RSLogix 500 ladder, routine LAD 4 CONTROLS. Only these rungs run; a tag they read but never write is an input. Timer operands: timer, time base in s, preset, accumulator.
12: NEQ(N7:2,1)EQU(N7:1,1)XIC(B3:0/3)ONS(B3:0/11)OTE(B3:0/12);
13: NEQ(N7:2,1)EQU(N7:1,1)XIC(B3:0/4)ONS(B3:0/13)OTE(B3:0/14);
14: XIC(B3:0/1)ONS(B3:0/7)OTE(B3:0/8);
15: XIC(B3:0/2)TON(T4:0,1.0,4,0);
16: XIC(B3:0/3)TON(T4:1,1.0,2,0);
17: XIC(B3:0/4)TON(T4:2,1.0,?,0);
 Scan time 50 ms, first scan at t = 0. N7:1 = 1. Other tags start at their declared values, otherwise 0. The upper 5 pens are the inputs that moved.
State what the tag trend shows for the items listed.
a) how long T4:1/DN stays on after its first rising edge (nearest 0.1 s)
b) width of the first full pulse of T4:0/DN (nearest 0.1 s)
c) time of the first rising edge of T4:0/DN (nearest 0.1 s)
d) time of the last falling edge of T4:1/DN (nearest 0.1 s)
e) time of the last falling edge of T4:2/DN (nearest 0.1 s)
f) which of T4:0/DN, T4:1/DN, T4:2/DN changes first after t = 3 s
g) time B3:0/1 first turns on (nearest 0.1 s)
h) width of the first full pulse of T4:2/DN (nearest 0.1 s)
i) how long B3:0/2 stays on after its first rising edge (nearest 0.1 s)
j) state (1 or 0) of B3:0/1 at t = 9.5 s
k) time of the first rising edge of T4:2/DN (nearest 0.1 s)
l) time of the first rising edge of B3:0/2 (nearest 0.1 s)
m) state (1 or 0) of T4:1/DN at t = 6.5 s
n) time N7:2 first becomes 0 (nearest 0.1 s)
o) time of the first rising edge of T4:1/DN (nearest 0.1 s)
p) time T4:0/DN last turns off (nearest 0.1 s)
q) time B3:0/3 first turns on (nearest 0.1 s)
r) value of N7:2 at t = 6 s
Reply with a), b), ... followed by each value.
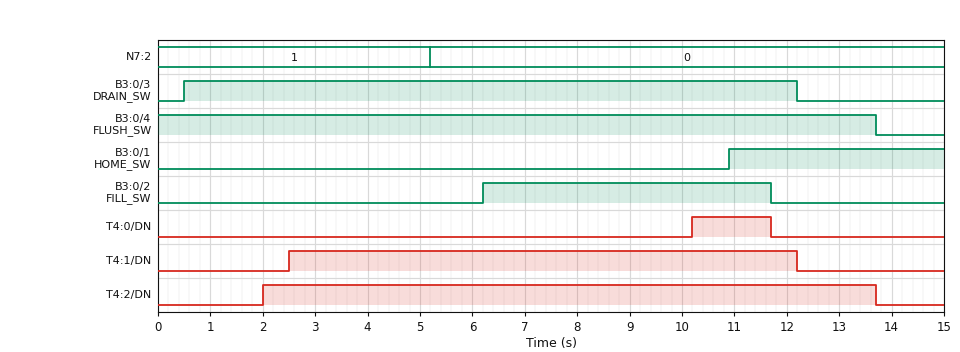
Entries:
a) 9.7 s
b) 1.5 s
c) 10.2 s
d) 12.2 s
e) 13.7 s
f) T4:0/DN
g) 10.9 s
h) 11.7 s
i) 5.5 s
j) 0
k) 2.0 s
l) 6.2 s
m) 1
n) 5.2 s
o) 2.5 s
p) 11.7 s
q) 0.5 s
r) 0
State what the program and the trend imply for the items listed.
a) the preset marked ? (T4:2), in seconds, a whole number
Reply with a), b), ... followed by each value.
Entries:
a) 2 s
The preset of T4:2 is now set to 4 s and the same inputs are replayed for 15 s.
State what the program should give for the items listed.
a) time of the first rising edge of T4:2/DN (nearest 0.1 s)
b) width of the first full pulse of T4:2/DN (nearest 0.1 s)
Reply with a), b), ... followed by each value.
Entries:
a) 4.0 s
b) 9.7 s
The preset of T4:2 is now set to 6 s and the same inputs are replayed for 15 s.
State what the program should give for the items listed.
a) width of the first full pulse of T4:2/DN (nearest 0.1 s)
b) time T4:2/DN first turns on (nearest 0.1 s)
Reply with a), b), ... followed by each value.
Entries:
a) 7.7 s
b) 6.0 s
